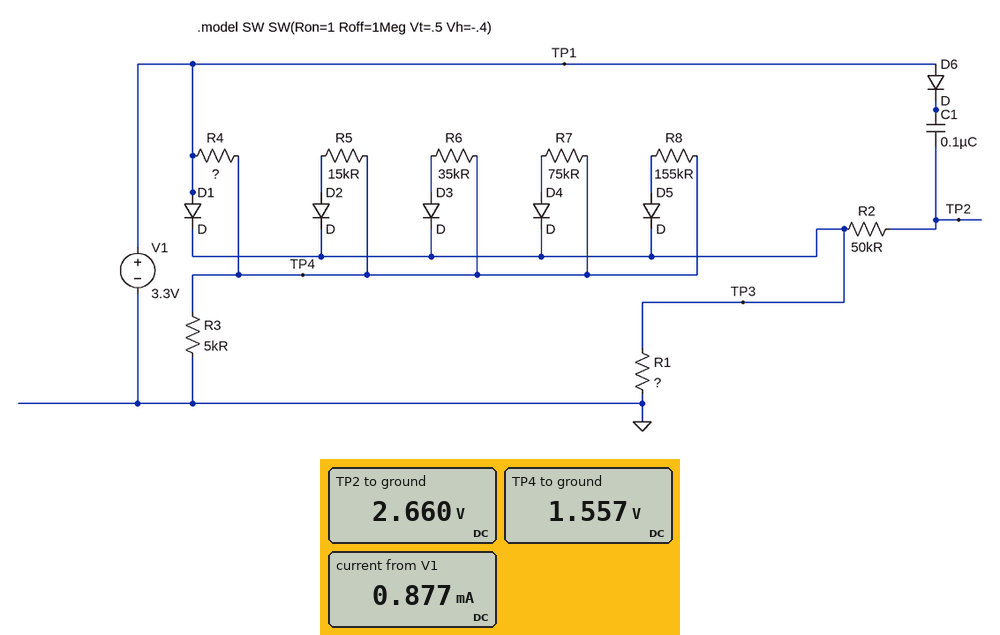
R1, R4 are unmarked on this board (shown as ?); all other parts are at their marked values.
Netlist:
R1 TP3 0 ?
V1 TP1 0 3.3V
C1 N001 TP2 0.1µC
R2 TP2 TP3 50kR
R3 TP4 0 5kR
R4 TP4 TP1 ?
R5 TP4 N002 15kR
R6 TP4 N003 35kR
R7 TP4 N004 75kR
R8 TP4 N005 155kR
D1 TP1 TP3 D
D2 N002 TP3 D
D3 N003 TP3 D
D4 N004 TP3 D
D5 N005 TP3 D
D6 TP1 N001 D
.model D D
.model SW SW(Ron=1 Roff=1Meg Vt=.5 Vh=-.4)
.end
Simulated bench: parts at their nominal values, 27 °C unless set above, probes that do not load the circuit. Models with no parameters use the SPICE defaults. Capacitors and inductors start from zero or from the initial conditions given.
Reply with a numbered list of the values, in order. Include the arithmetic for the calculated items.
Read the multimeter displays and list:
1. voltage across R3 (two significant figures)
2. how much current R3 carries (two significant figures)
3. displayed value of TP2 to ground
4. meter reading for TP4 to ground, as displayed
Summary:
1. 1.557 V = 1.6 V
2. (1.557 V) / 5 kΩ = 310 µA
3. 2.660 V
4. 1.557 V
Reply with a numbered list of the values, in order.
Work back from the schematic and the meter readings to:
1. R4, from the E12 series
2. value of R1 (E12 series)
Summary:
1. 5.6 kΩ
2. 4.7 kΩ
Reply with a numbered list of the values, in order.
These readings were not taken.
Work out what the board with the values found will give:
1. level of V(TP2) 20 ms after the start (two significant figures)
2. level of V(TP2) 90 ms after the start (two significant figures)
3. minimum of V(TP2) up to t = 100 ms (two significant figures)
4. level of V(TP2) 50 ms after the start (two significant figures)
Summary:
1. 2.7 V
2. 2.7 V
3. 2.7 V
4. 2.7 V
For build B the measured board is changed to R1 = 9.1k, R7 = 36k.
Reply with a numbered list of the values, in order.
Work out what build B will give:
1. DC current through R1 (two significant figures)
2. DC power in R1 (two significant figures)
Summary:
1. 290 µA
2. 790 µW
